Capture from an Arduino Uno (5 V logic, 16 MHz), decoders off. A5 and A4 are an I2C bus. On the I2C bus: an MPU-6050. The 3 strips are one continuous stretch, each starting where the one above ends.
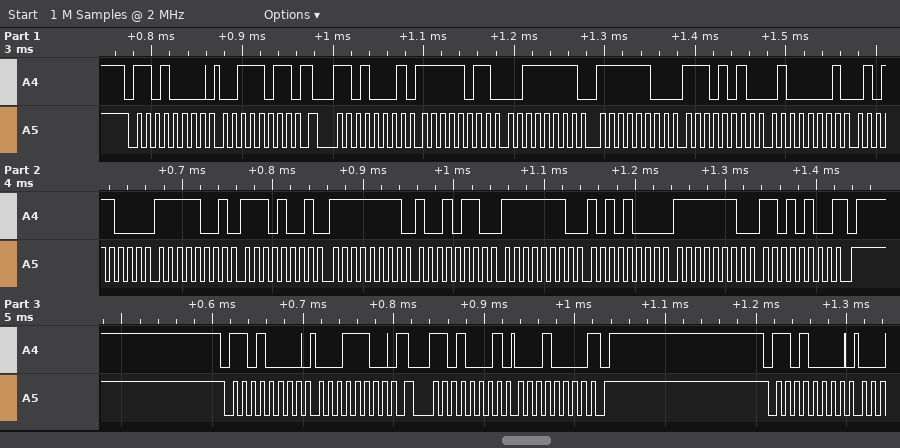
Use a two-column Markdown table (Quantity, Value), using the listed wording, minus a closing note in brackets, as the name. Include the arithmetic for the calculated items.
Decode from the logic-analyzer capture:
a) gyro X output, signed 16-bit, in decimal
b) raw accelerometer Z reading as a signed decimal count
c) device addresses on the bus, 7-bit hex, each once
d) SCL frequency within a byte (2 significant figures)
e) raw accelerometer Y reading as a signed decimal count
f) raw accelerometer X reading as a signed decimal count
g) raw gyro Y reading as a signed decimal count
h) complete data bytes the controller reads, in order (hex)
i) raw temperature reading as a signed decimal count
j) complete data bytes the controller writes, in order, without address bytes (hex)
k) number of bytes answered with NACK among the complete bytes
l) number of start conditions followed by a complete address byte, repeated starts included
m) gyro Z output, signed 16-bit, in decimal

| Quantity | Value |
|---|---|
| gyro X output, signed 16-bit, in decimal | 0xFF96 = -106 |
| raw accelerometer Z reading as a signed decimal count | 0x4158 = 16728 |
| device addresses on the bus, 7-bit hex, each once | 0x68 |
| SCL frequency within a byte | 100 kHz |
| raw accelerometer Y reading as a signed decimal count | 0xFCEA = -790 |
| raw accelerometer X reading as a signed decimal count | 0xFB3F = -1217 |
| raw gyro Y reading as a signed decimal count | 0xFEA8 = -344 |
| complete data bytes the controller reads, in order | FB 3F FC EA 41 58 F9 E9 FF 96 FE A8 FE D4 10 |
| raw temperature reading as a signed decimal count | 0xF9E9 = -1559 |
| complete data bytes the controller writes, in order, without address bytes | 3B 1C |
| number of bytes answered with NACK among the complete bytes | 2 |
| number of start conditions followed by a complete address byte, repeated starts included | 5 |
| gyro Z output, signed 16-bit, in decimal | 0xFED4 = -300 |
